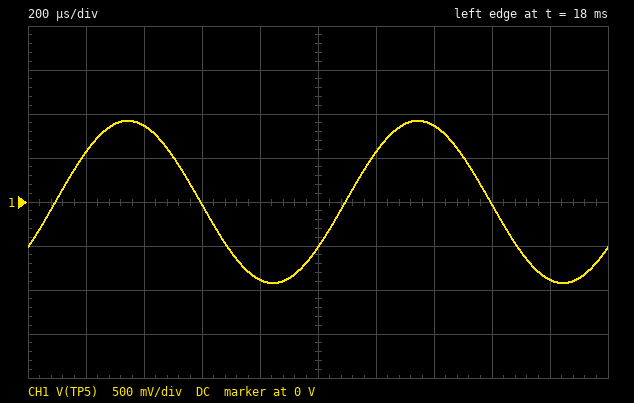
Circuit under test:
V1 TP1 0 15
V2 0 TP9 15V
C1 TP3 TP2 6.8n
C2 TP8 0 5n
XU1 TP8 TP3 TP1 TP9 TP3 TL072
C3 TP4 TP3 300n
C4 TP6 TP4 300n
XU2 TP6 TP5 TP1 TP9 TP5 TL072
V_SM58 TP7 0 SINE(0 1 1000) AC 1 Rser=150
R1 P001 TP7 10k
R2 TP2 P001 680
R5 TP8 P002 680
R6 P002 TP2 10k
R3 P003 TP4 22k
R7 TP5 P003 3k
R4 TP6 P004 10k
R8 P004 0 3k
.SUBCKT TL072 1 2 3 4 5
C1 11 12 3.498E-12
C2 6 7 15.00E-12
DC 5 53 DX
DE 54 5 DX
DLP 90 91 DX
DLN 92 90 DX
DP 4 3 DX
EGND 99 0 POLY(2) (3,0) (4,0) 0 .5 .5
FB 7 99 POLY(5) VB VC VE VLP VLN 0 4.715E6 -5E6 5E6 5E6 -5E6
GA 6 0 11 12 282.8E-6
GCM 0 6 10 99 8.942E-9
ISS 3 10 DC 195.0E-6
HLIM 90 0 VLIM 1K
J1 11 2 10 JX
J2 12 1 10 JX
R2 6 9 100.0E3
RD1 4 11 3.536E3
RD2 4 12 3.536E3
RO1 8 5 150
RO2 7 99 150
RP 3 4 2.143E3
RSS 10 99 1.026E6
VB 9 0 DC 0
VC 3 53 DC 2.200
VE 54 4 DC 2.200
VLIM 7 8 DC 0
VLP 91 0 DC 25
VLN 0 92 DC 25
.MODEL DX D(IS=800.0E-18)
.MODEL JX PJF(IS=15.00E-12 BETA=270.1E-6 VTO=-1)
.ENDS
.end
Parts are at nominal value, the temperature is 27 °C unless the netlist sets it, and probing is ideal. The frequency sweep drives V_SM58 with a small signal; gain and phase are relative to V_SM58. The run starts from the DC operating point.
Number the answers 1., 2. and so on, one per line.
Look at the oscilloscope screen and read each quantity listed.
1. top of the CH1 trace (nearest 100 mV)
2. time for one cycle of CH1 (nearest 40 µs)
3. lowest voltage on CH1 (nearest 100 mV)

1. 900 mV
2. 1.00 ms
3. -900 mV
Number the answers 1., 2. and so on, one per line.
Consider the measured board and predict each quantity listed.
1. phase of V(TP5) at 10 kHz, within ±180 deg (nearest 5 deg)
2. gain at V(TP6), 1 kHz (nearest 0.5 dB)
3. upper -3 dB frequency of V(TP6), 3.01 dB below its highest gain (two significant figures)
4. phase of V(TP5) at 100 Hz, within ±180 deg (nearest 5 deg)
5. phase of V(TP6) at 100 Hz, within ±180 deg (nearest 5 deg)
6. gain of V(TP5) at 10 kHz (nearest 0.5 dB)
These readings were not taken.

1. -155 deg
2. -0.5 dB
3. 2.1 kHz
4. 40 deg
5. 40 deg
6. -24.0 dB
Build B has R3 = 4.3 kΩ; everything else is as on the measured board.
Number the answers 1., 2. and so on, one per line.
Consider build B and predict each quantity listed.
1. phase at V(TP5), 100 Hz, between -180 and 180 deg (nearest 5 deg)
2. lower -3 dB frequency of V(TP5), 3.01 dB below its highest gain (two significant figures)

1. 45 deg
2. 57 Hz
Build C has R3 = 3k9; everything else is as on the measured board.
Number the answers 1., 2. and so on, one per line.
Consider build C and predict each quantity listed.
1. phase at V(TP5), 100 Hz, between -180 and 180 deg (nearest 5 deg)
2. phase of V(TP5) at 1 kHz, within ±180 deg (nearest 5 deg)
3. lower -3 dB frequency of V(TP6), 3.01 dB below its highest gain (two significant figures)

1. 45 deg
2. -35 deg
3. 57 Hz
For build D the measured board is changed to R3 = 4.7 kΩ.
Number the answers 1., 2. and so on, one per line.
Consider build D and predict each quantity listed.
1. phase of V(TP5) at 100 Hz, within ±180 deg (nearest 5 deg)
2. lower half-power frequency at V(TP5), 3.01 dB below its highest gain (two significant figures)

1. 45 deg
2. 57 Hz
